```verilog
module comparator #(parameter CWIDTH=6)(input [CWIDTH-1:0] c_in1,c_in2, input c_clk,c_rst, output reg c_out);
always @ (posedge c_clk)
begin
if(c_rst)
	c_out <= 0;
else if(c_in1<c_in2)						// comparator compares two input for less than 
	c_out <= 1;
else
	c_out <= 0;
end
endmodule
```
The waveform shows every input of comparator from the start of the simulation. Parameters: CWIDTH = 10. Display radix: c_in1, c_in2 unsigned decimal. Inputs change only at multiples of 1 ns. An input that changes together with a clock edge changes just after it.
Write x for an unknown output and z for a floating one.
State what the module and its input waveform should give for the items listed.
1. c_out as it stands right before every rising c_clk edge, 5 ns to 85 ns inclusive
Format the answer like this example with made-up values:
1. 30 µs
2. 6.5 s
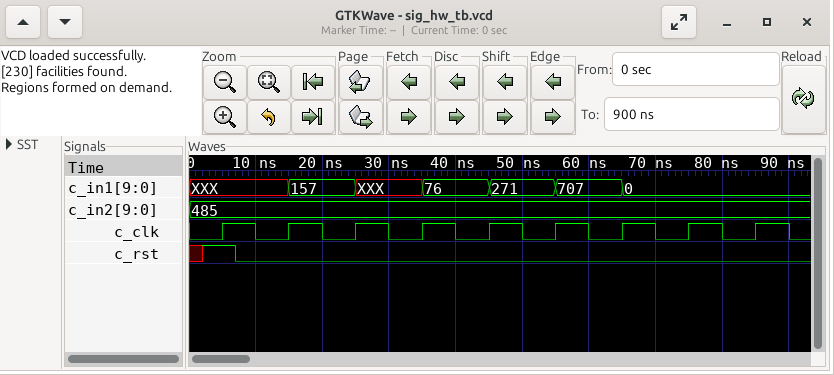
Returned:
1. x 0 0 1 0 1 1 0 1
